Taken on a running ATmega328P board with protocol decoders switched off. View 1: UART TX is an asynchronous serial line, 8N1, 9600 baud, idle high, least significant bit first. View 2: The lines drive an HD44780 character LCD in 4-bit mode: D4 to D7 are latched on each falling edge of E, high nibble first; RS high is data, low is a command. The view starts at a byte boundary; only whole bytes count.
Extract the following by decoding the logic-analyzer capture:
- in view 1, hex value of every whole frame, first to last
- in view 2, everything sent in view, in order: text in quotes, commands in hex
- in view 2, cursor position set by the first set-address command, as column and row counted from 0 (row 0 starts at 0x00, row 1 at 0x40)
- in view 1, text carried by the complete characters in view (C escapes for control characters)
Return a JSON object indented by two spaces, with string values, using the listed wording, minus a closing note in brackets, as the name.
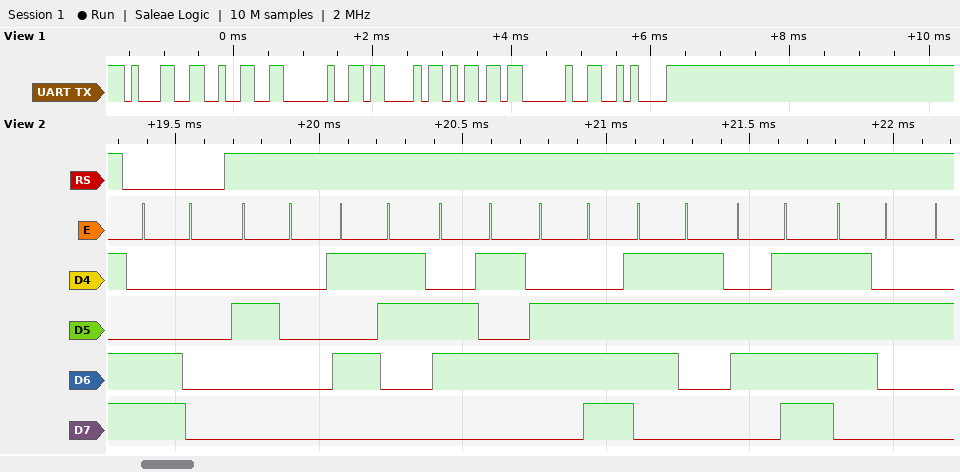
{
  "in view 1, hex value of every whole frame, first to last": "31 32 20 43 6D 20 0A",
  "in view 2, everything sent in view, in order: text in quotes, commands in hex": "0xC0 \" Sensor\"",
  "in view 2, cursor position set by the first set-address command, as column and row counted from 0": "column 0, row 1",
  "in view 1, text carried by the complete characters in view": "\"12 Cm \\n\""
}
